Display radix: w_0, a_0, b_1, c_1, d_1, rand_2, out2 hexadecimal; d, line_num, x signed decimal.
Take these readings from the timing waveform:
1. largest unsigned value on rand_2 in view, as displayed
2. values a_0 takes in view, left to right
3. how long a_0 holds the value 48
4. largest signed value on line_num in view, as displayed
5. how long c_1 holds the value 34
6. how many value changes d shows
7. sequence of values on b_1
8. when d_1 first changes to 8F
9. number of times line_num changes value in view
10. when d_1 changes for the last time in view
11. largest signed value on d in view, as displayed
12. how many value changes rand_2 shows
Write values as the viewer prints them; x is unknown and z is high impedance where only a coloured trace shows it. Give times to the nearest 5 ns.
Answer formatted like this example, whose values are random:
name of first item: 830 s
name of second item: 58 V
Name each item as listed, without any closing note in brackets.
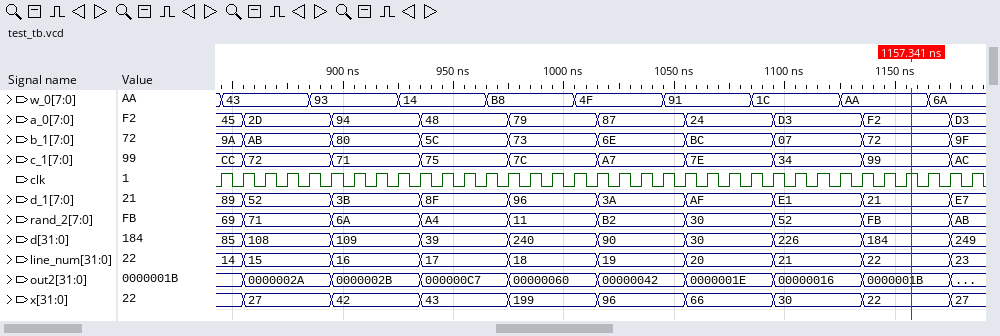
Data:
largest unsigned value on rand_2 in view, as displayed: FB
values a_0 takes in view, left to right: 45, 2D, 94, 48, 79, 87, 24, D3, F2, D3
how long a_0 holds the value 48: 40 ns
largest signed value on line_num in view, as displayed: 23
how long c_1 holds the value 34: 40 ns
how many value changes d shows: 9
sequence of values on b_1: 9A, AB, 80, 5C, 73, 6E, BC, 07, 72, 9F
when d_1 first changes to 8F: 935 ns
number of times line_num changes value in view: 9
when d_1 changes for the last time in view: 1175 ns
largest signed value on d in view, as displayed: 249
how many value changes rand_2 shows: 9
